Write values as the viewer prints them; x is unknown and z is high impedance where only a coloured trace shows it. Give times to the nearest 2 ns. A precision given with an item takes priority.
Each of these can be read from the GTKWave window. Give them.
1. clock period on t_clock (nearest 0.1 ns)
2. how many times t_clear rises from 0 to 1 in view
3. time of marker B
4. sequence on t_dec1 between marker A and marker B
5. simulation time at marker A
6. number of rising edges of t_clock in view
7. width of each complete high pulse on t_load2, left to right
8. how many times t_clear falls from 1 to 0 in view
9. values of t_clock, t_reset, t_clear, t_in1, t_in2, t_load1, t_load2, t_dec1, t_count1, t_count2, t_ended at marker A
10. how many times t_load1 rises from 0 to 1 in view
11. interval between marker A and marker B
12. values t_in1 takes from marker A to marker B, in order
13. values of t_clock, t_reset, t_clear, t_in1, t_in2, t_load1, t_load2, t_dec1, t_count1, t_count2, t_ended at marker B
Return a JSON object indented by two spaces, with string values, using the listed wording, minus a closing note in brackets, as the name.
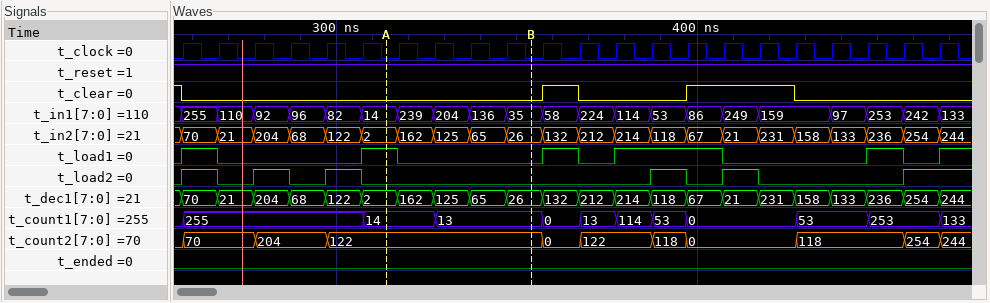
{
  "clock period on t_clock": "10 ns",
  "how many times t_clear rises from 0 to 1 in view": "2",
  "time of marker B": "354 ns",
  "sequence on t_dec1 between marker A and marker B": "2, 162, 125, 65, 26",
  "simulation time at marker A": "314 ns",
  "number of rising edges of t_clock in view": "22",
  "width of each complete high pulse on t_load2, left to right": "10 ns, 10 ns, 10 ns, 10 ns, 10 ns",
  "how many times t_clear falls from 1 to 0 in view": "3",
  "values of t_clock, t_reset, t_clear, t_in1, t_in2, t_load1, t_load2, t_dec1, t_count1, t_count2, t_ended at marker A": "t_clock=0, t_reset=1, t_clear=0, t_in1=14, t_in2=2, t_load1=1, t_load2=0, t_dec1=2, t_count1=14, t_count2=122, t_ended=0",
  "how many times t_load1 rises from 0 to 1 in view": "6",
  "interval between marker A and marker B": "40 ns",
  "values t_in1 takes from marker A to marker B, in order": "14, 239, 204, 136, 35",
  "values of t_clock, t_reset, t_clear, t_in1, t_in2, t_load1, t_load2, t_dec1, t_count1, t_count2, t_ended at marker B": "t_clock=0, t_reset=1, t_clear=0, t_in1=35, t_in2=26, t_load1=0, t_load2=0, t_dec1=26, t_count1=13, t_count2=122, t_ended=0"
}
